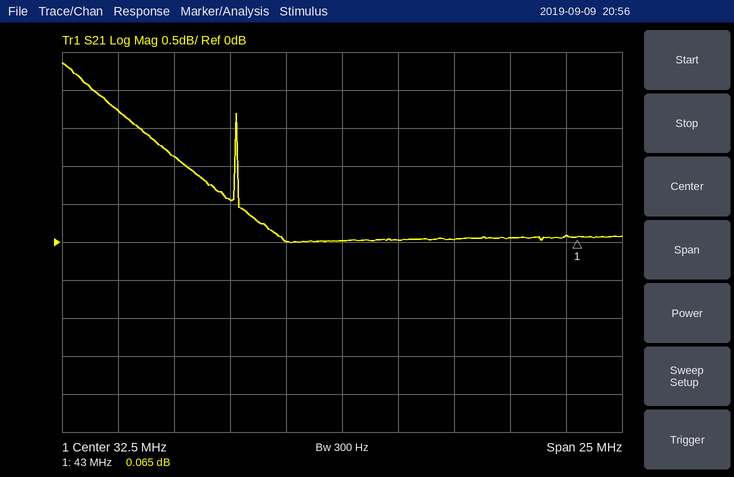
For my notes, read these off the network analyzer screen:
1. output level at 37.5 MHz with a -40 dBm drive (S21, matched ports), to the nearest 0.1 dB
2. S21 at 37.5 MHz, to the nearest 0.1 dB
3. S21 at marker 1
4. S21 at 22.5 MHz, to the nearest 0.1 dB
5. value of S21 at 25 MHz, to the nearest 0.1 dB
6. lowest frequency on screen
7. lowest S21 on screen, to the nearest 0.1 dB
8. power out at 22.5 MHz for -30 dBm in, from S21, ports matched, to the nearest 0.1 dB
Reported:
-40.0 dBm
0.0 dB
0.065 dB
1.7 dB
1.1 dB
20 MHz
0.0 dB
-28.3 dBm
